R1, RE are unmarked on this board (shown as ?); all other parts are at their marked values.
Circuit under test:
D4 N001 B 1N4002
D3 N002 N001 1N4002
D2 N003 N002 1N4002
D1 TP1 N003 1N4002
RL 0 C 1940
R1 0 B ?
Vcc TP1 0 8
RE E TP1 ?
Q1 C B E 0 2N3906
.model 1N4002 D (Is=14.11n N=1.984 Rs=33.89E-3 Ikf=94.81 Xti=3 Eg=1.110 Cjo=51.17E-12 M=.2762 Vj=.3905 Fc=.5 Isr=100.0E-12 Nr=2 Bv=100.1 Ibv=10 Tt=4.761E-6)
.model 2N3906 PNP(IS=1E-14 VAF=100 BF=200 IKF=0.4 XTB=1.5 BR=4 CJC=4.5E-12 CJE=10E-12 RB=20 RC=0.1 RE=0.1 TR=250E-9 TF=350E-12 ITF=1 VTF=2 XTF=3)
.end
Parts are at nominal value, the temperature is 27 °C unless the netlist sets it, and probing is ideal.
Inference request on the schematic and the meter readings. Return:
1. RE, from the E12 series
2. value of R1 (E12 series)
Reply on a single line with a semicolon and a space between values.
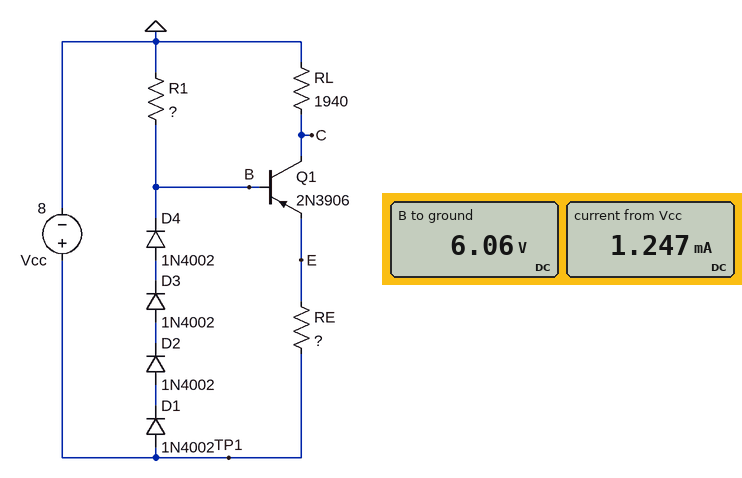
1.2 kΩ; 33 kΩ
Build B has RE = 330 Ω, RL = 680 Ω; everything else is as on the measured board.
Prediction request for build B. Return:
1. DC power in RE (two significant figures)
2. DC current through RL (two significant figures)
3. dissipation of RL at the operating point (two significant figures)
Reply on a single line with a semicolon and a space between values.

4.6 mW; 3.7 mA; 9.4 mW
